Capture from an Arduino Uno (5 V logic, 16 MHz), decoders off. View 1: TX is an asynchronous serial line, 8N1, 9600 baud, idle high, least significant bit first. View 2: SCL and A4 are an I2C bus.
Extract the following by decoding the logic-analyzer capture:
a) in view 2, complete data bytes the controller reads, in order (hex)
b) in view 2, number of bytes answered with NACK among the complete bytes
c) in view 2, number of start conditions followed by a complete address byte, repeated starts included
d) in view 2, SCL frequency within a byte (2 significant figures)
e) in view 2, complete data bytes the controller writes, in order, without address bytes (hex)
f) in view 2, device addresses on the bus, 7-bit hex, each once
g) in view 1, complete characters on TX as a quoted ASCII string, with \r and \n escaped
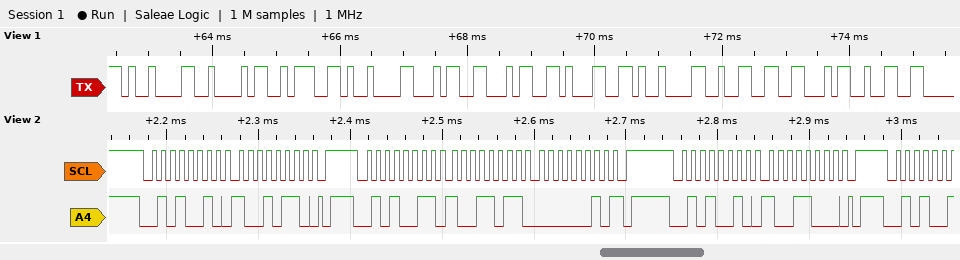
9B 02
1
3
100 kHz
96 98
0x29
"\tB:\t441\t2F2"
